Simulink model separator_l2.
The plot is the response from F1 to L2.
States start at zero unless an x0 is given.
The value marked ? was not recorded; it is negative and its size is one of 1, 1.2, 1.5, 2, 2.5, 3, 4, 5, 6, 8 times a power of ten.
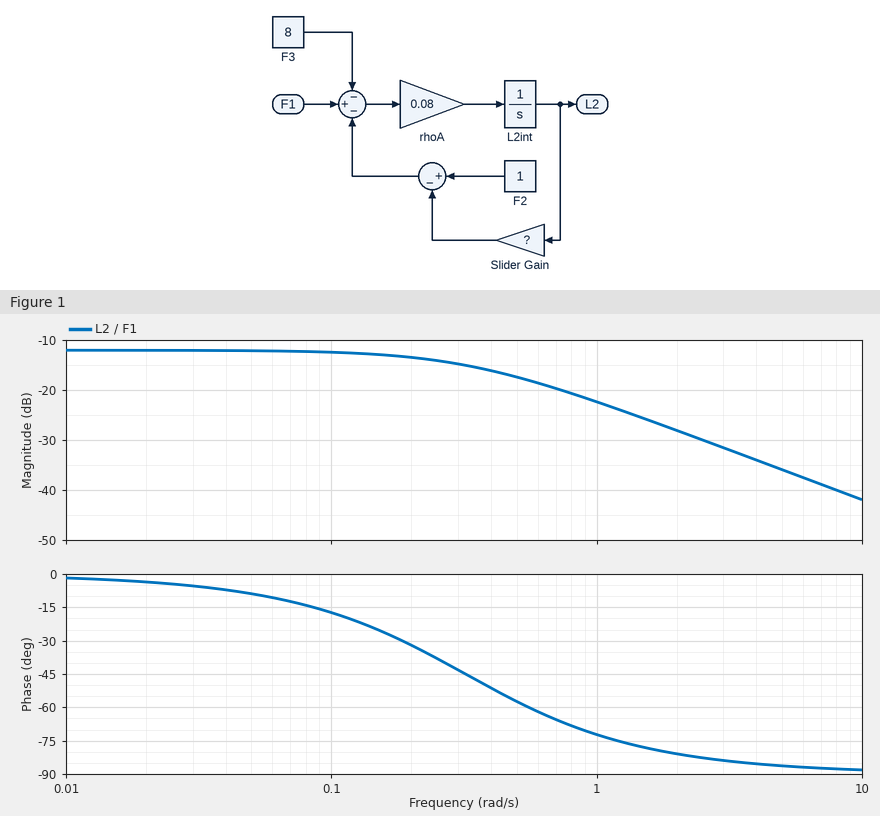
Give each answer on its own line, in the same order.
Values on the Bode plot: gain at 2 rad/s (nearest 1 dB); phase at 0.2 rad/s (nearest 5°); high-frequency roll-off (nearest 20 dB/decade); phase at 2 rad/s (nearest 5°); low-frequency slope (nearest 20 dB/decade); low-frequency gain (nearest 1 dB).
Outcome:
-28 dB
-30°
-20 dB/decade
-80°
0 dB/decade
-12 dB
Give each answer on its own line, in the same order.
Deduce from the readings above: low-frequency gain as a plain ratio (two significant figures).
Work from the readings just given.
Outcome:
0.25
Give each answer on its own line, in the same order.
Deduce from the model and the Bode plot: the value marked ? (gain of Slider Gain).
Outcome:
-4
